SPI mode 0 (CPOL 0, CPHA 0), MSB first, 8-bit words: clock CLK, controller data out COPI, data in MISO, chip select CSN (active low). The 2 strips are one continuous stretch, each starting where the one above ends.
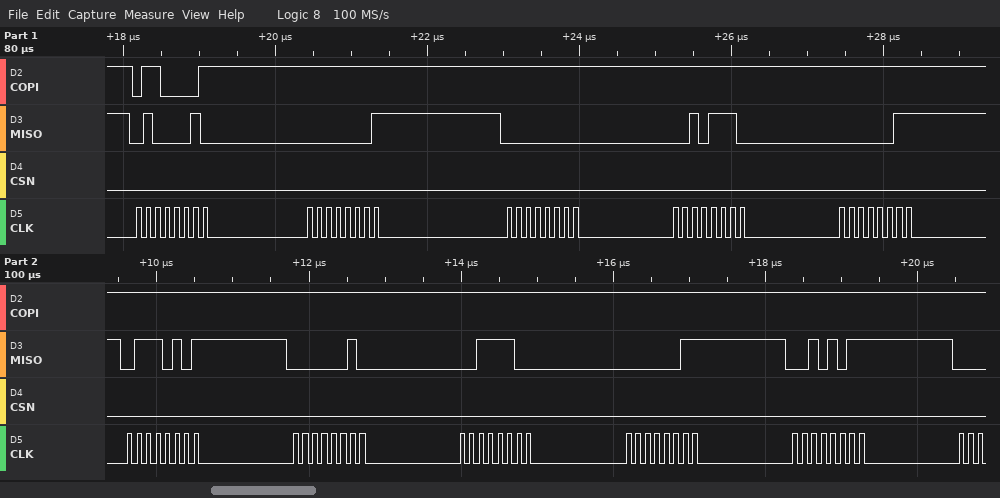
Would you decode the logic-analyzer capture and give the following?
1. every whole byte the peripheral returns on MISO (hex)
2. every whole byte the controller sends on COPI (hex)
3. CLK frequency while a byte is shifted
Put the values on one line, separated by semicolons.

42 01 00 2E 03 75 02 3C 03 2B; 61 FF FF FF FF FF FF FF FF FF; 8 MHz
